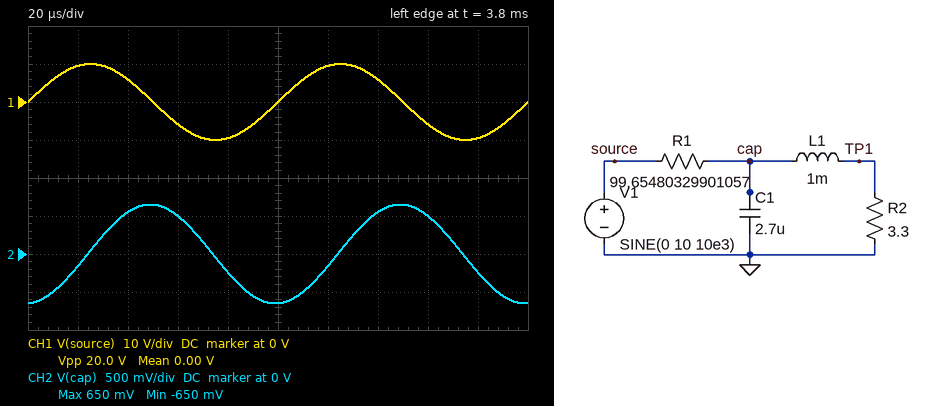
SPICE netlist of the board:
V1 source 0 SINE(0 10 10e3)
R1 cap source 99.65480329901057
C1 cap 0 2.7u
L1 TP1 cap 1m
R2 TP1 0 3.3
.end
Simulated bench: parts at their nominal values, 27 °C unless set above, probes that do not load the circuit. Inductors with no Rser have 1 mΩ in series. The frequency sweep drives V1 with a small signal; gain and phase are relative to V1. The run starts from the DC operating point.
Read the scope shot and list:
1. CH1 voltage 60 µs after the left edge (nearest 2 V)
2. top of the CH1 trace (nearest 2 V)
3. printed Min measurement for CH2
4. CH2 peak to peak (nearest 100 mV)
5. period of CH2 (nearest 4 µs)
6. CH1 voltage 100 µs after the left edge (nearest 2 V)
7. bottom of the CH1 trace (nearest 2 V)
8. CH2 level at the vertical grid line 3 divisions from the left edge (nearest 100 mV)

-6 V
10 V
-650 mV
1.3 V
100 µs
0 V
-10 V
500 mV
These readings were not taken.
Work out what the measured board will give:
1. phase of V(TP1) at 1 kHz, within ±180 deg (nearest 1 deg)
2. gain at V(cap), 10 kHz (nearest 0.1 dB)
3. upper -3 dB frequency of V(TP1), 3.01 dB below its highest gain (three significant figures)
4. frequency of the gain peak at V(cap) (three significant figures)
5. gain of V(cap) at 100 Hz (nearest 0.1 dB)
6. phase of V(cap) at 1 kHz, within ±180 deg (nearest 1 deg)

-7 deg
-23.7 dB
3.53 kHz
3.11 kHz
-29.7 dB
55 deg
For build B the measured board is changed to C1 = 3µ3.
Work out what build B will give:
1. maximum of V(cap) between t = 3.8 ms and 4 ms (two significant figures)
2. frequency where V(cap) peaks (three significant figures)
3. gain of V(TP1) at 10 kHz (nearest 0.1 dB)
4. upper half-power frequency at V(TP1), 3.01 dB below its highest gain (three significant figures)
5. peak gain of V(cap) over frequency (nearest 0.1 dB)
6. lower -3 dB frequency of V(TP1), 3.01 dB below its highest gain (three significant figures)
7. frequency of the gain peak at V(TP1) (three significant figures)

520 mV
2.81 kHz
-51.2 dB
3.20 kHz
-6.2 dB
2.15 kHz
2.72 kHz
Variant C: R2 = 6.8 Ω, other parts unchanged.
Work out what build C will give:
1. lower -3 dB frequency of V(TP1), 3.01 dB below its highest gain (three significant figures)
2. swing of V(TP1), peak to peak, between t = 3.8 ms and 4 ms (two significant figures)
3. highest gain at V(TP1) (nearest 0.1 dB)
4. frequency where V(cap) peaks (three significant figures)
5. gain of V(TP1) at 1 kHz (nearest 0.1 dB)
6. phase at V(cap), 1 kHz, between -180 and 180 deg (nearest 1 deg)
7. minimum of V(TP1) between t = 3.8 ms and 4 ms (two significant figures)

1.87 kHz
140 mV
-18.0 dB
3.14 kHz
-23.1 dB
32 deg
-70 mV
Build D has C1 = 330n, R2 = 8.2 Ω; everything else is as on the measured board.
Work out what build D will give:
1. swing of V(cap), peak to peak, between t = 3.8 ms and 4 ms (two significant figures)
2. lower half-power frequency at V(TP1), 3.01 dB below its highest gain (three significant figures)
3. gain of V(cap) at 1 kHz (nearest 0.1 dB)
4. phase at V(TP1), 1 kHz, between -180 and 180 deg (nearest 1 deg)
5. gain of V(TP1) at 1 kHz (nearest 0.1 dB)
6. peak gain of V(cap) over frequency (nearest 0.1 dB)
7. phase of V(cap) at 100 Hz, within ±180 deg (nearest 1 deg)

15 V
3.39 kHz
-20.3 dB
-4 deg
-22.3 dB
-2.0 dB
4 deg
